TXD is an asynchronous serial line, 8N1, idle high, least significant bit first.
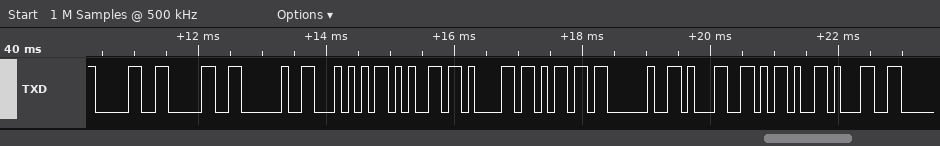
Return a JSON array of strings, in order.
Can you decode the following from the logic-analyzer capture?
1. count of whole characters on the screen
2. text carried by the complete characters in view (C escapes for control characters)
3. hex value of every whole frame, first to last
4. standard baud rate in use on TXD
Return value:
["11", "\"00 Team 1-1\"", "0x30 0x30 0x20 0x54 0x65 0x61 0x6D 0x20 0x31 0x2D 0x31", "9600 baud"]
